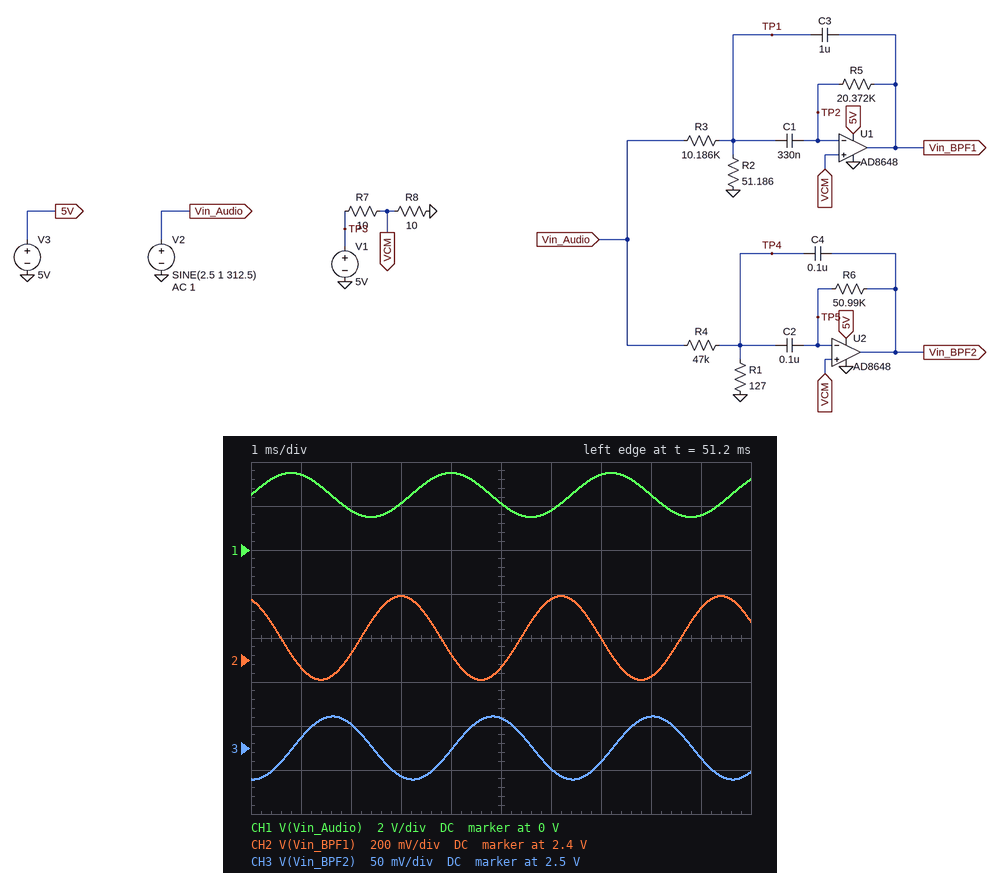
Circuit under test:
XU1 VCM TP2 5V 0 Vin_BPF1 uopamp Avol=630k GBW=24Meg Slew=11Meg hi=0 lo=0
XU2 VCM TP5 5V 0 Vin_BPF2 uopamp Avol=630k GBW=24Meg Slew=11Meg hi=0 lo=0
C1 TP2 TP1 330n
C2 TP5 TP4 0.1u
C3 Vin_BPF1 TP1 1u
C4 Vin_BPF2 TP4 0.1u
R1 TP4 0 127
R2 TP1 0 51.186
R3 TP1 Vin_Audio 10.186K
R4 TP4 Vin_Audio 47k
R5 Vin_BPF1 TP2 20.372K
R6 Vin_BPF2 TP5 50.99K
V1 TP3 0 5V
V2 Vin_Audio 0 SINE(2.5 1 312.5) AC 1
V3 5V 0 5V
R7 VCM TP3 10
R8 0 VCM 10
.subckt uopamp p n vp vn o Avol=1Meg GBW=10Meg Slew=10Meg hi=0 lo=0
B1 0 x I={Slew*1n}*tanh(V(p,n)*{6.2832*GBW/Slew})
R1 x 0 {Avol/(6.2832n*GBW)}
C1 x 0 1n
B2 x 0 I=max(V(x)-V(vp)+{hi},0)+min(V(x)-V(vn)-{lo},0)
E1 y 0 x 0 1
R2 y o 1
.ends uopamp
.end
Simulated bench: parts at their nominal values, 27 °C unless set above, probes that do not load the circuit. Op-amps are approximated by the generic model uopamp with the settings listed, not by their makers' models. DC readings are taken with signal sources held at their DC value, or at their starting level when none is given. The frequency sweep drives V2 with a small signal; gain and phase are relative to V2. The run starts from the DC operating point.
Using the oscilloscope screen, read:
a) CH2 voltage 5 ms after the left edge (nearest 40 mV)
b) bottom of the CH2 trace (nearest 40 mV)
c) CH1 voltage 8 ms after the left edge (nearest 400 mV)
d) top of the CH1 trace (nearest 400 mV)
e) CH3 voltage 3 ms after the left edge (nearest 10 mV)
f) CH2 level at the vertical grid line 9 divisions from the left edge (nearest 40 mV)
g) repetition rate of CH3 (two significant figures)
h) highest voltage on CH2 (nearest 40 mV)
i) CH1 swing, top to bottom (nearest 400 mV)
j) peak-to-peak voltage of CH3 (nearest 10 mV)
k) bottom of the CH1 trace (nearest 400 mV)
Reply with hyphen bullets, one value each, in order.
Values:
- 2.36 V
- 2.32 V
- 2.4 V
- 3.6 V
- 2.47 V
- 2.64 V
- 310 Hz
- 2.68 V
- 2.0 V
- 70 mV
- 1.6 V
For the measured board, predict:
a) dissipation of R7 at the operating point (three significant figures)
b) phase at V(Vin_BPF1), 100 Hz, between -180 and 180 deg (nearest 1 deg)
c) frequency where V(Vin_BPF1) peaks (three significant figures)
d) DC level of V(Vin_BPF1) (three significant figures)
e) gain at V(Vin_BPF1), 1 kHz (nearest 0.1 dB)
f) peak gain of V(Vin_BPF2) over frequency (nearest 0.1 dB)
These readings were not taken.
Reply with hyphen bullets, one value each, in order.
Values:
- 625 mW
- -93 deg
- 272 Hz
- 2.50 V
- -35.5 dB
- -5.3 dB
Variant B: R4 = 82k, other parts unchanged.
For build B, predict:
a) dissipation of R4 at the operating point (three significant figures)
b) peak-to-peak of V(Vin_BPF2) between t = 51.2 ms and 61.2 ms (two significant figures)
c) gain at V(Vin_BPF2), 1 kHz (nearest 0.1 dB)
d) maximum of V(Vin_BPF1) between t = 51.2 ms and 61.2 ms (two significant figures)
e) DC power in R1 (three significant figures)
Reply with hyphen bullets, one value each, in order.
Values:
- 76.0 µW
- 41 mV
- -30.0 dB
- 2.7 V
- 118 nW
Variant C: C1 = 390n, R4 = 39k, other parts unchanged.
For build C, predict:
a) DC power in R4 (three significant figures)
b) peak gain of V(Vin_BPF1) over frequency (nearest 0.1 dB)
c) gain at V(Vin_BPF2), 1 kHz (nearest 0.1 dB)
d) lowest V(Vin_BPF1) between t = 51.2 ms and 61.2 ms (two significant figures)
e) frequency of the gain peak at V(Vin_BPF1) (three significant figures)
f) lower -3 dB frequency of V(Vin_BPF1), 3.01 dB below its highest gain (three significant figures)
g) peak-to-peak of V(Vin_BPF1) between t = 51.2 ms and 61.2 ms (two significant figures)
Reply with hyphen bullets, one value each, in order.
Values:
- 159 µW
- -5.0 dB
- -23.5 dB
- 2.4 V
- 250 Hz
- 237 Hz
- 270 mV
